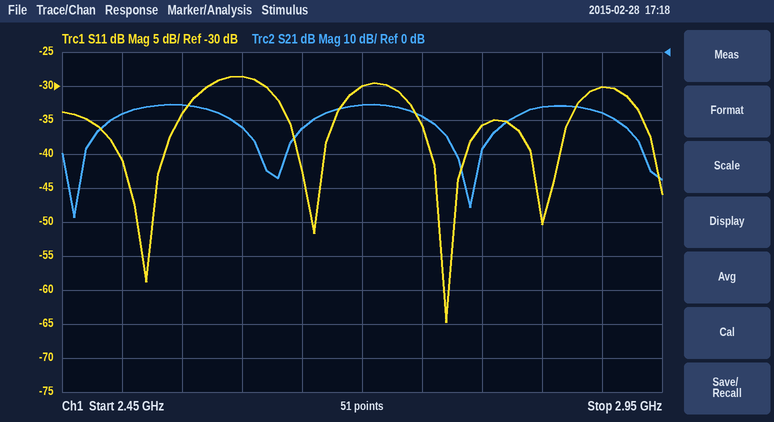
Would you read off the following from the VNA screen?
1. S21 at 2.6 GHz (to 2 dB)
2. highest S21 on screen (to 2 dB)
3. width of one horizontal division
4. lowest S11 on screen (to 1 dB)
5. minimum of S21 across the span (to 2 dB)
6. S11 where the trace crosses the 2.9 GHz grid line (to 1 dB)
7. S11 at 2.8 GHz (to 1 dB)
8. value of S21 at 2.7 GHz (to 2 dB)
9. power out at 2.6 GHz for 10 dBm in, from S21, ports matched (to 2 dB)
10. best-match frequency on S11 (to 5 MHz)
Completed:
-22 dB
-16 dB
50 MHz
-65 dB
-48 dB
-30 dB
-36 dB
-16 dB
-12 dBm
2.770 GHz
